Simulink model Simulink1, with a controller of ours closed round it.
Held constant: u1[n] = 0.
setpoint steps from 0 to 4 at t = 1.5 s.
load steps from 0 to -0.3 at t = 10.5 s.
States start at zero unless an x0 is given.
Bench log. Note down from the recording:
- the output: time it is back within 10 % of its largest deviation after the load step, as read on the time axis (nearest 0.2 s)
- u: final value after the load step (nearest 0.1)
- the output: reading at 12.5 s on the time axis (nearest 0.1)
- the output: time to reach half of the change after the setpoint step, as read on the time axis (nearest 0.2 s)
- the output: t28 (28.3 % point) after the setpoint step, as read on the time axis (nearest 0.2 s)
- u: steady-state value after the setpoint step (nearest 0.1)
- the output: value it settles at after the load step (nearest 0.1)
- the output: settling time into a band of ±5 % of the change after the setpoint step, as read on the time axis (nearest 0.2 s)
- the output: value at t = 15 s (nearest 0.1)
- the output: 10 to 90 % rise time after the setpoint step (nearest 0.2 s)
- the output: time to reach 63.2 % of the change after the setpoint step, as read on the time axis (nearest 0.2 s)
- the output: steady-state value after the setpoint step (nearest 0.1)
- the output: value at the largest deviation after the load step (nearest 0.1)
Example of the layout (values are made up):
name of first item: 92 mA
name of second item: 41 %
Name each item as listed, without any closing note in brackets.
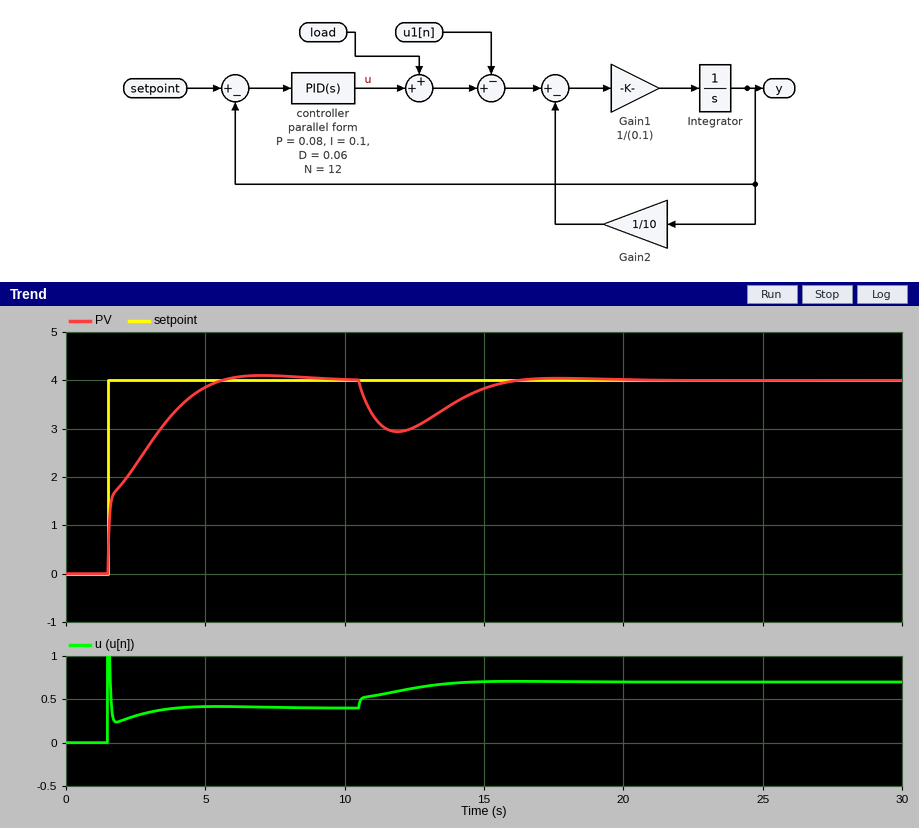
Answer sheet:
the output: time it is back within 10 % of its largest deviation after the load step, as read on the time axis: 15.4 s
u: final value after the load step: 0.7
the output: reading at 12.5 s on the time axis: 3.0
the output: time to reach half of the change after the setpoint step, as read on the time axis: 2.2 s
the output: t28 (28.3 % point) after the setpoint step, as read on the time axis: 1.6 s
u: steady-state value after the setpoint step: 0.4
the output: value it settles at after the load step: 4.0
the output: settling time into a band of ±5 % of the change after the setpoint step, as read on the time axis: 4.8 s
the output: value at t = 15 s: 3.8
the output: 10 to 90 % rise time after the setpoint step: 2.8 s
the output: time to reach 63.2 % of the change after the setpoint step, as read on the time axis: 2.8 s
the output: steady-state value after the setpoint step: 4.0
the output: value at the largest deviation after the load step: 2.9
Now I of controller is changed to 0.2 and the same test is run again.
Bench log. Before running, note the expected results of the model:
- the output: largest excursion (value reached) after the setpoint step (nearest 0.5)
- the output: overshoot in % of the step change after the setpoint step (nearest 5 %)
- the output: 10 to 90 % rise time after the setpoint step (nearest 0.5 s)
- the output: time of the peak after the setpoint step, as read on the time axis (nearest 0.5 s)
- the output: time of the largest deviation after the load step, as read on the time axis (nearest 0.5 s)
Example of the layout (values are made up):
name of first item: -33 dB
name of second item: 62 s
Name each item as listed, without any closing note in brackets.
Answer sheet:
the output: largest excursion (value reached) after the setpoint step: 4.5
the output: overshoot in % of the step change after the setpoint step: 10 %
the output: 10 to 90 % rise time after the setpoint step: 1.5 s
the output: time of the peak after the setpoint step, as read on the time axis: 4.5 s
the output: time of the largest deviation after the load step, as read on the time axis: 11.5 s
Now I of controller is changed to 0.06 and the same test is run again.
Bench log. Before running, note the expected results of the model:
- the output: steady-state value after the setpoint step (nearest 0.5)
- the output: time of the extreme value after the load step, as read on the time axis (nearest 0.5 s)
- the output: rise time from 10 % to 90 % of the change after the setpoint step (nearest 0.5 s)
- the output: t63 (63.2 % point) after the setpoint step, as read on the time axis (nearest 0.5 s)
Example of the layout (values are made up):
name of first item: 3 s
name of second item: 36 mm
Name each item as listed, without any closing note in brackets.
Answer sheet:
the output: steady-state value after the setpoint step: 4.0
the output: time of the extreme value after the load step, as read on the time axis: 12.0 s
the output: rise time from 10 % to 90 % of the change after the setpoint step: 4.5 s
the output: t63 (63.2 % point) after the setpoint step, as read on the time axis: 3.5 s
